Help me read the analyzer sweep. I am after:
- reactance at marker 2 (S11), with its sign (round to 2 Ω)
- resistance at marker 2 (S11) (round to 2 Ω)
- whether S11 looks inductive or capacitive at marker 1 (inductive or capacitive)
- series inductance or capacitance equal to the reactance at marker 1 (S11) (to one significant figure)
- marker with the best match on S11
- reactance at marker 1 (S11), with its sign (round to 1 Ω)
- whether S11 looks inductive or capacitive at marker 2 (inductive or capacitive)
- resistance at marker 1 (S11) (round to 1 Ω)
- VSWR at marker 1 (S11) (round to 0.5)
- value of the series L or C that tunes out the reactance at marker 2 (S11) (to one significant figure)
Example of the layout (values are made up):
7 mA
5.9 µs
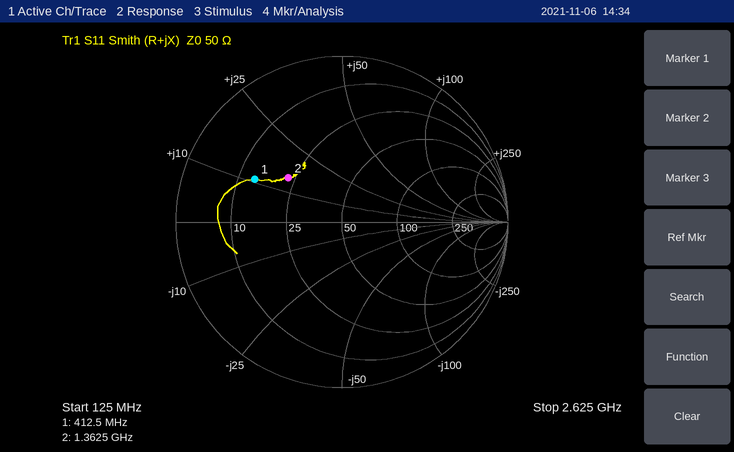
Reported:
+14 Ω
22 Ω
inductive
4 nH
marker 2
+11 Ω
inductive
14 Ω
4.0
8 pF
